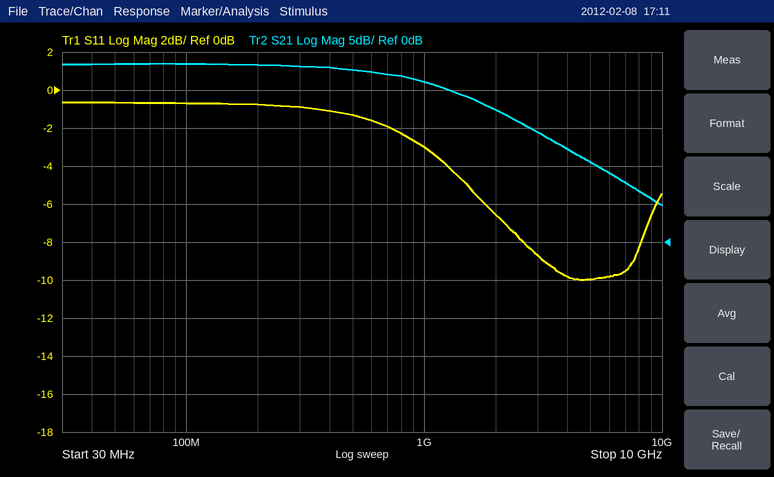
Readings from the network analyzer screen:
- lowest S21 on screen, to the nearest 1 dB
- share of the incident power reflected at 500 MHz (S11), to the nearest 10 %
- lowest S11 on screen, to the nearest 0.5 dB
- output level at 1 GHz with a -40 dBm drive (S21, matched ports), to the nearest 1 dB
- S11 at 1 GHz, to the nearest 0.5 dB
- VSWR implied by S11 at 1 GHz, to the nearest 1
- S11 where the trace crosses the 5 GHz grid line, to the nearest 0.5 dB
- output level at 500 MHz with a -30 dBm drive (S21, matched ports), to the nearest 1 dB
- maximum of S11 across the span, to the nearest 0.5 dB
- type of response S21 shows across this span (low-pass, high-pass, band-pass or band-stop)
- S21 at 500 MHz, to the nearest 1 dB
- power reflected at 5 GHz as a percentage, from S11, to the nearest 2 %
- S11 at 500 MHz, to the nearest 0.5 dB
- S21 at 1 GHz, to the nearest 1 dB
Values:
5 dB
70 %
-10.0 dB
-19 dBm
-3.0 dB
6
-10.0 dB
-7 dBm
-0.5 dB
low-pass
23 dB
10 %
-1.5 dB
21 dB
